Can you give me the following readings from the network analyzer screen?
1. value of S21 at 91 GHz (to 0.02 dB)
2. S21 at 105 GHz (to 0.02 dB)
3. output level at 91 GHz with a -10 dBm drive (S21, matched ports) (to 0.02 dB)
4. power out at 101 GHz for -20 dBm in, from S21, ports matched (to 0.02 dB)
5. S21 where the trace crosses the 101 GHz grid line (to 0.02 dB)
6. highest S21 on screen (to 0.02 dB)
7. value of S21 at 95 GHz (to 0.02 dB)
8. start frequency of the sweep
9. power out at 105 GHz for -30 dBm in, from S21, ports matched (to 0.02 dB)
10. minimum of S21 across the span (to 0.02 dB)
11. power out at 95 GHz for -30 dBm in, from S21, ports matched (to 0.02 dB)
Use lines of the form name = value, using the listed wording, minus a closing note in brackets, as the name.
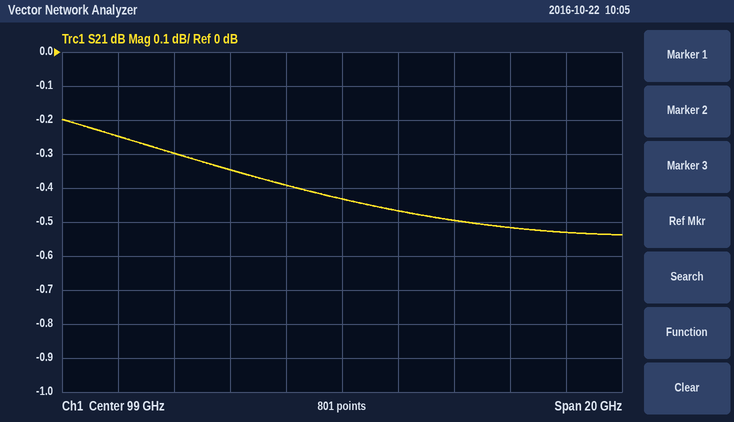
value of S21 at 91 GHz = -0.24 dB
S21 at 105 GHz = -0.52 dB
output level at 91 GHz with a -10 dBm drive (S21, matched ports) = -10.24 dBm
power out at 101 GHz for -20 dBm in, from S21, ports matched = -20.46 dBm
S21 where the trace crosses the 101 GHz grid line = -0.46 dB
highest S21 on screen = -0.20 dB
value of S21 at 95 GHz = -0.34 dB
start frequency of the sweep = 89 GHz
power out at 105 GHz for -30 dBm in, from S21, ports matched = -30.52 dBm
minimum of S21 across the span = -0.54 dB
power out at 95 GHz for -30 dBm in, from S21, ports matched = -30.34 dBm
